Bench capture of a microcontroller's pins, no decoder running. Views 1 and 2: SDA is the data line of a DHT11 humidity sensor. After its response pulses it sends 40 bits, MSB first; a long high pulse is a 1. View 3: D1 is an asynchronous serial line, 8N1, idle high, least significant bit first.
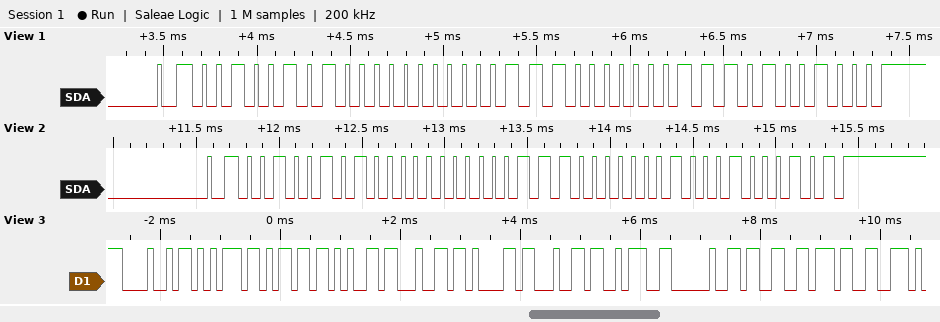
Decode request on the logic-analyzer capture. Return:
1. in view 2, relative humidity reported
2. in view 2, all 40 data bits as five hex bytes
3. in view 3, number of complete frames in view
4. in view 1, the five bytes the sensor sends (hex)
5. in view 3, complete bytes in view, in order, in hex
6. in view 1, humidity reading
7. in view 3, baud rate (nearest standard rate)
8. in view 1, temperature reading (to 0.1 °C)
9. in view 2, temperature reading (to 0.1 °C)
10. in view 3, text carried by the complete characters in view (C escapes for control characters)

37 %
25 00 1C 04 45
11
25 00 1C 07 48
48 75 6D 65 64 61 64 3A 20 33 37
37 %
9600 baud
28.7 °C
28.4 °C
"Humedad: 37"
